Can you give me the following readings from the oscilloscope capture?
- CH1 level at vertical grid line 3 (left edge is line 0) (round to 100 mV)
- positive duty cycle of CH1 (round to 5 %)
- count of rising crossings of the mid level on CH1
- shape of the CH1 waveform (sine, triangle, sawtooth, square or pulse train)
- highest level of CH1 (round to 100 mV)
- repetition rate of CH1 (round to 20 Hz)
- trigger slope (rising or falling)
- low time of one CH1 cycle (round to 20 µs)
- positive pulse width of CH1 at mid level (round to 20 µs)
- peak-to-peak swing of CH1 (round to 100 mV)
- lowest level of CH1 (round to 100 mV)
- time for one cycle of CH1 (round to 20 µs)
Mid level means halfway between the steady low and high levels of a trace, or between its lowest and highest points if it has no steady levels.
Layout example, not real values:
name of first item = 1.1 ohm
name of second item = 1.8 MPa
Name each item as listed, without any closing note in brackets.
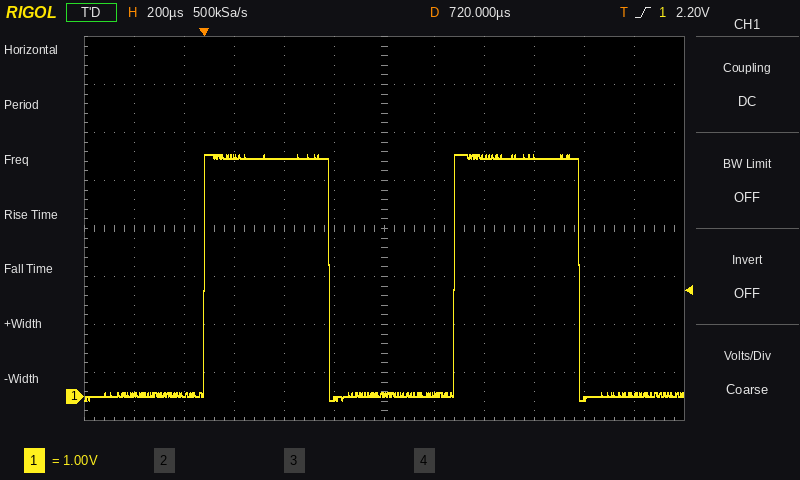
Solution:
CH1 level at vertical grid line 3 (left edge is line 0) = 5.0 V
positive duty cycle of CH1 = 50 %
count of rising crossings of the mid level on CH1 = 2
shape of the CH1 waveform = square
highest level of CH1 = 5.0 V
repetition rate of CH1 = 1.00 kHz
trigger slope = rising
low time of one CH1 cycle = 500 µs
positive pulse width of CH1 at mid level = 500 µs
peak-to-peak swing of CH1 = 5.1 V
lowest level of CH1 = -100 mV
time for one cycle of CH1 = 1.00 ms
